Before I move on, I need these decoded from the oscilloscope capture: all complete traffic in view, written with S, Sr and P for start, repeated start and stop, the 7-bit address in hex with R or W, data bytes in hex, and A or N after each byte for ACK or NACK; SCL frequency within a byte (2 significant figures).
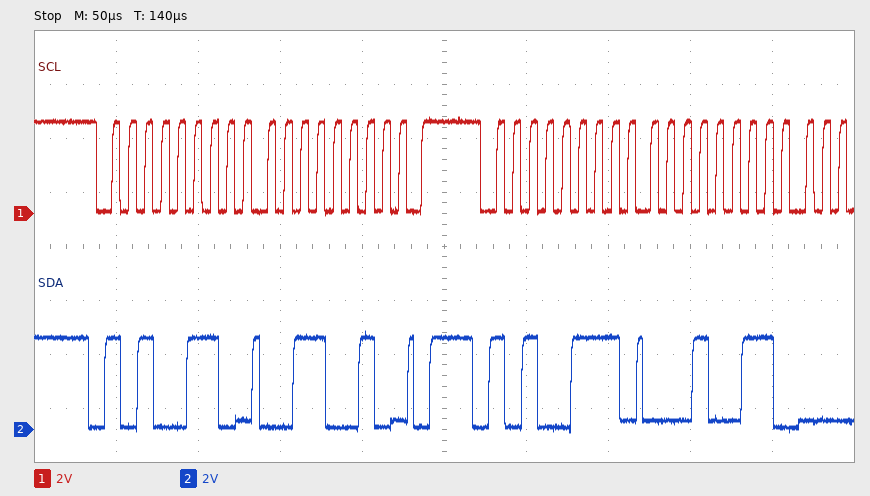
S 53W A 32 A P S 53R A 13 A
100 kHz
